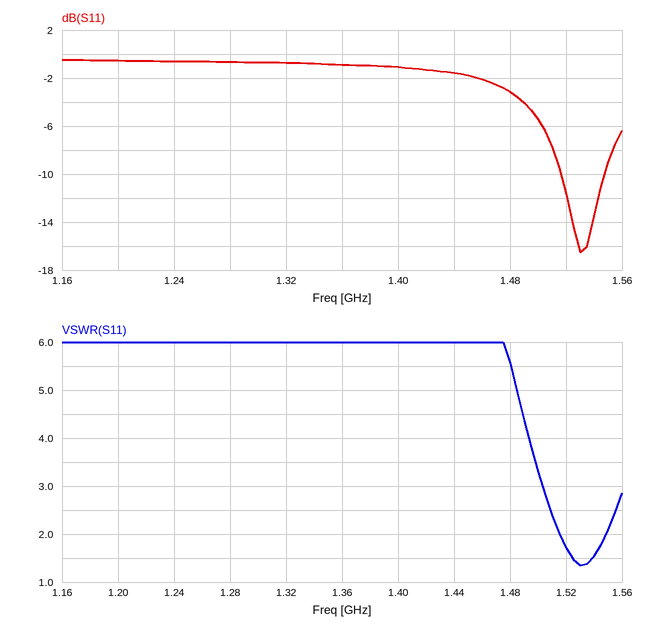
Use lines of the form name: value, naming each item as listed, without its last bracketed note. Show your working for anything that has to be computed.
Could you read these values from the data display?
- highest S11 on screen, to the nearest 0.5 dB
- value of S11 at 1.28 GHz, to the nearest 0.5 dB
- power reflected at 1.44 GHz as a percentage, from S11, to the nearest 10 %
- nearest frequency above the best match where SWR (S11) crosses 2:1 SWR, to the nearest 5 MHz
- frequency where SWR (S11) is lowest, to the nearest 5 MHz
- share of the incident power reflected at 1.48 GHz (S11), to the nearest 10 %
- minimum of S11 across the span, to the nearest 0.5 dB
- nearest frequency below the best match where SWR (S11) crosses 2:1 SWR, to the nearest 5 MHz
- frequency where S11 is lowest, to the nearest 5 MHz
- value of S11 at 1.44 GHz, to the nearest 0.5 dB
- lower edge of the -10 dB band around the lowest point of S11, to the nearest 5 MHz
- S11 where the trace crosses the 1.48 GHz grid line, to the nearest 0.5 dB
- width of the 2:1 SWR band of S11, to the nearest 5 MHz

highest S11 on screen, to the nearest 0.5 dB: -0.5 dB
value of S11 at 1.28 GHz, to the nearest 0.5 dB: -0.5 dB
power reflected at 1.44 GHz as a percentage, from S11, to the nearest 10 %: 10^(-1.5/10) ≈ 70.8 %, so 70 % to the nearest 10 %
nearest frequency above the best match where SWR (S11) crosses 2:1 SWR, to the nearest 5 MHz: 1.550 GHz
frequency where SWR (S11) is lowest, to the nearest 5 MHz: 1.530 GHz
share of the incident power reflected at 1.48 GHz (S11), to the nearest 10 %: 10^(-3/10) ≈ 50 %
minimum of S11 across the span, to the nearest 0.5 dB: -16.5 dB
nearest frequency below the best match where SWR (S11) crosses 2:1 SWR, to the nearest 5 MHz: 1.515 GHz
frequency where S11 is lowest, to the nearest 5 MHz: 1.530 GHz
value of S11 at 1.44 GHz, to the nearest 0.5 dB: -1.5 dB
lower edge of the -10 dB band around the lowest point of S11, to the nearest 5 MHz: 1.515 GHz
S11 where the trace crosses the 1.48 GHz grid line, to the nearest 0.5 dB: -3.0 dB
width of the 2:1 SWR band of S11, to the nearest 5 MHz: 1.550 GHz − 1.515 GHz = 35 MHz
